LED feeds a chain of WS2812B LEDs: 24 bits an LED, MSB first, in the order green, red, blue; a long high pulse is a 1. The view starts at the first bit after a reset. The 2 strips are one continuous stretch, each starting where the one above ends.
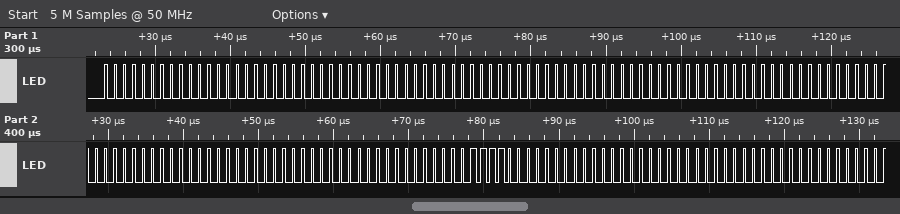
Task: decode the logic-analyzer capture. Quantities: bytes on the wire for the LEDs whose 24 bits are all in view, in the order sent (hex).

00 00 00 00 00 00 00 00 00 00 00 00 00 00 00 0F 00 00 00 00 00
